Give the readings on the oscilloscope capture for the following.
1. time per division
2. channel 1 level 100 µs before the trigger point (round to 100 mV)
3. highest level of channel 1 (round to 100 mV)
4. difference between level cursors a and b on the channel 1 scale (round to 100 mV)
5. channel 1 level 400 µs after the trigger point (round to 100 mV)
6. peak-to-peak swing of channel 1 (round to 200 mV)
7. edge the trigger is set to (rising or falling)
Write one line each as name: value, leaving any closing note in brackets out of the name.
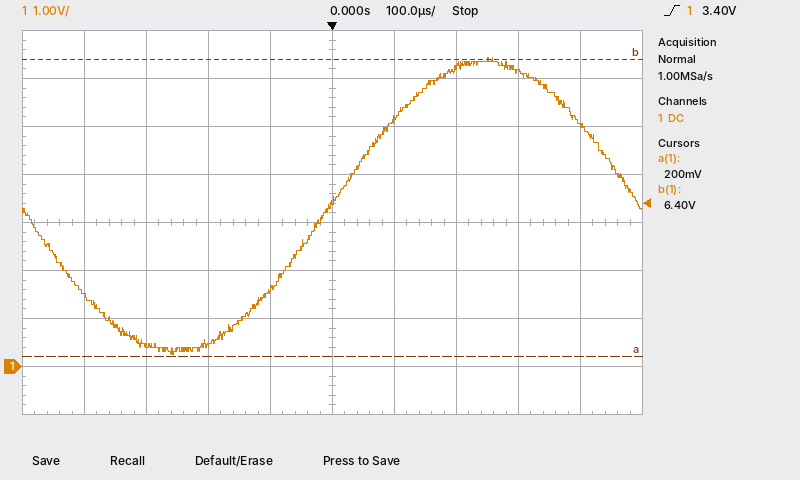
time per division: 100 µs
channel 1 level 100 µs before the trigger point: 1.6 V
highest level of channel 1: 6.4 V
difference between level cursors a and b on the channel 1 scale: 6.2 V
channel 1 level 400 µs after the trigger point: 5.1 V
peak-to-peak swing of channel 1: 6.2 V
edge the trigger is set to: rising
